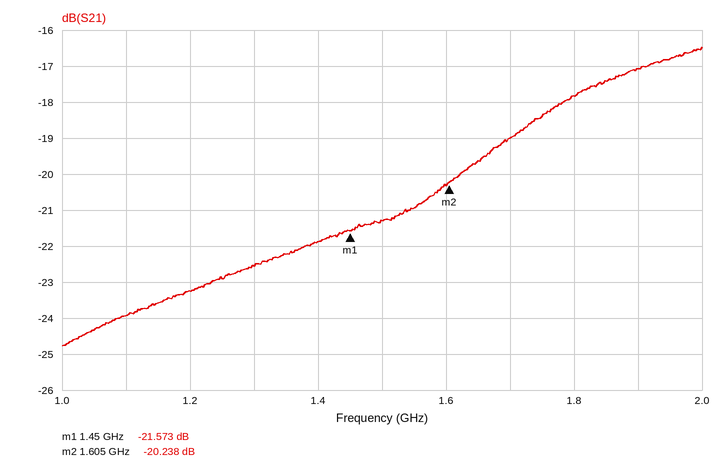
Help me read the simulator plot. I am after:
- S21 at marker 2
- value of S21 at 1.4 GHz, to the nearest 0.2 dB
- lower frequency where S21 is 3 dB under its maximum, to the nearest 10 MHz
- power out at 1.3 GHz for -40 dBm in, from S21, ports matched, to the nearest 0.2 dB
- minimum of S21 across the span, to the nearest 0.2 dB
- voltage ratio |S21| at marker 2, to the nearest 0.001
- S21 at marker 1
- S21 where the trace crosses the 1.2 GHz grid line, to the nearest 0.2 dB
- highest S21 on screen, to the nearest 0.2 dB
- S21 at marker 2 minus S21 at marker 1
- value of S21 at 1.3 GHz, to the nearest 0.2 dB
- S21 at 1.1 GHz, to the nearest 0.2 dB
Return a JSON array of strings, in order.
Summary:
["-20.238 dB", "-21.8 dB", "1.66 GHz", "-62.6 dBm", "-24.8 dB", "0.097", "-21.573 dB", "-23.2 dB", "-16.4 dB", "1.335 dB", "-22.6 dB", "-24.0 dB"]
